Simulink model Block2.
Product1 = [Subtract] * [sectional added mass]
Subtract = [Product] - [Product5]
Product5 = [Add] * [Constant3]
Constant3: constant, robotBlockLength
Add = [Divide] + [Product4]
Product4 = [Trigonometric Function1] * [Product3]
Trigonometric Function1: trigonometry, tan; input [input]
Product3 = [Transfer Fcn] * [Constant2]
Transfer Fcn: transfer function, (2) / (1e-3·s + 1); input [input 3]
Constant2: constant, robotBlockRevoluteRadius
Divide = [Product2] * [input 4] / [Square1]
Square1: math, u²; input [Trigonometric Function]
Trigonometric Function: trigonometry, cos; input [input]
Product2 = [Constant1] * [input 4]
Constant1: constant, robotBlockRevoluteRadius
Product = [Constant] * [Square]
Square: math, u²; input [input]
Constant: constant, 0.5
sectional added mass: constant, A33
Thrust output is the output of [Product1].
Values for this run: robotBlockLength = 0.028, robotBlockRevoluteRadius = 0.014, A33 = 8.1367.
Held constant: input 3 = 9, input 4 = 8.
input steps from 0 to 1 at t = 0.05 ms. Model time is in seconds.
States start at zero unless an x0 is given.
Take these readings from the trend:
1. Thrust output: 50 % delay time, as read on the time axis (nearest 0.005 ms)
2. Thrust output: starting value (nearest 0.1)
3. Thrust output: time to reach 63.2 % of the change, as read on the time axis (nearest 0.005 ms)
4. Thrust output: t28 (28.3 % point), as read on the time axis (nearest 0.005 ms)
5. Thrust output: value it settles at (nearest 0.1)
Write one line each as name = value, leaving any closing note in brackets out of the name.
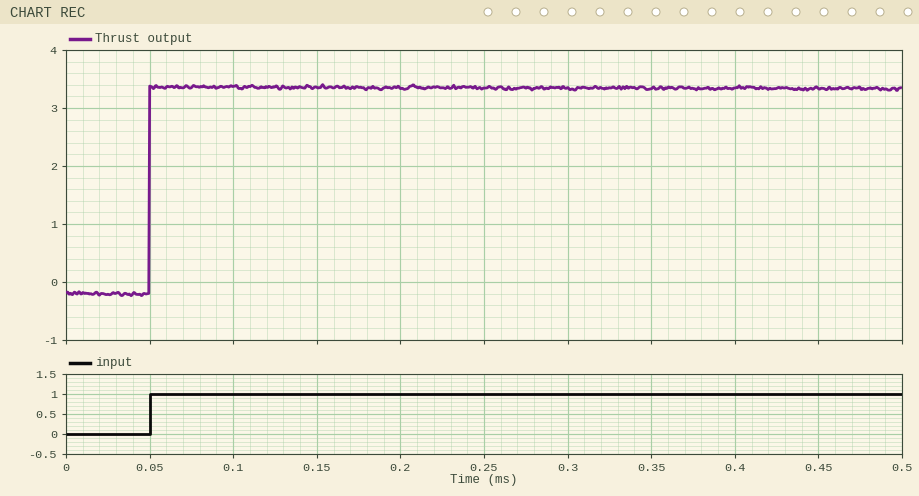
Thrust output: 50 % delay time, as read on the time axis = 0.050 ms
Thrust output: starting value = -0.2
Thrust output: time to reach 63.2 % of the change, as read on the time axis = 0.050 ms
Thrust output: t28 (28.3 % point), as read on the time axis = 0.050 ms
Thrust output: value it settles at = 3.3
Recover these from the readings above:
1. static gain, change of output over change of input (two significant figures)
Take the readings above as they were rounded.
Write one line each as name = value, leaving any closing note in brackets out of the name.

static gain, change of output over change of input = 3.5
